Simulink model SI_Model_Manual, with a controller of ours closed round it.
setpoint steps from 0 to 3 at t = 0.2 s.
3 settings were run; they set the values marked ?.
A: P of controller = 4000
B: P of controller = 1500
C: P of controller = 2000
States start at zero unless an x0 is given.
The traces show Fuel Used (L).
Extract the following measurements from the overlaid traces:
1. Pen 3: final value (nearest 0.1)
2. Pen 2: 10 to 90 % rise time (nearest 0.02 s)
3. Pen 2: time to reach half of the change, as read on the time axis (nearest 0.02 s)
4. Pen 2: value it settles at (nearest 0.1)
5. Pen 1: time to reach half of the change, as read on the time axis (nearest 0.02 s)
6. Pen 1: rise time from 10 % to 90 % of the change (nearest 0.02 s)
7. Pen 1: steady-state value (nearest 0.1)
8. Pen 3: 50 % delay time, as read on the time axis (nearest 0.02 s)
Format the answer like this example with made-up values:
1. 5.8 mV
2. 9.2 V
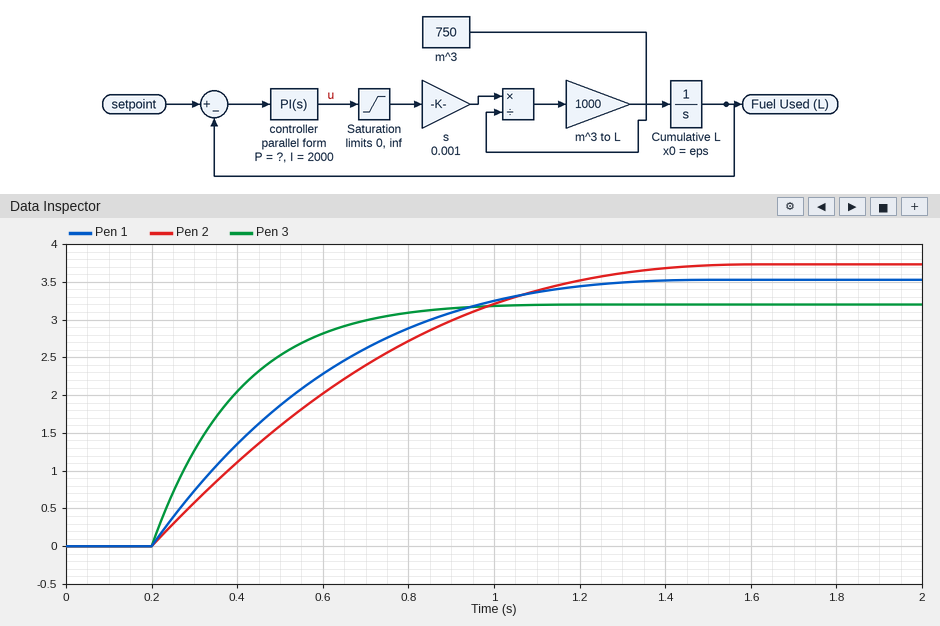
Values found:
1. 3.2
2. 0.82 s
3. 0.56 s
4. 3.7
5. 0.48 s
6. 0.70 s
7. 3.5
8. 0.34 s
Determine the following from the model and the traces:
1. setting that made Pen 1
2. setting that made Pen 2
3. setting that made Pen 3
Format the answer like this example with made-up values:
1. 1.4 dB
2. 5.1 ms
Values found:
1. C
2. B
3. A
